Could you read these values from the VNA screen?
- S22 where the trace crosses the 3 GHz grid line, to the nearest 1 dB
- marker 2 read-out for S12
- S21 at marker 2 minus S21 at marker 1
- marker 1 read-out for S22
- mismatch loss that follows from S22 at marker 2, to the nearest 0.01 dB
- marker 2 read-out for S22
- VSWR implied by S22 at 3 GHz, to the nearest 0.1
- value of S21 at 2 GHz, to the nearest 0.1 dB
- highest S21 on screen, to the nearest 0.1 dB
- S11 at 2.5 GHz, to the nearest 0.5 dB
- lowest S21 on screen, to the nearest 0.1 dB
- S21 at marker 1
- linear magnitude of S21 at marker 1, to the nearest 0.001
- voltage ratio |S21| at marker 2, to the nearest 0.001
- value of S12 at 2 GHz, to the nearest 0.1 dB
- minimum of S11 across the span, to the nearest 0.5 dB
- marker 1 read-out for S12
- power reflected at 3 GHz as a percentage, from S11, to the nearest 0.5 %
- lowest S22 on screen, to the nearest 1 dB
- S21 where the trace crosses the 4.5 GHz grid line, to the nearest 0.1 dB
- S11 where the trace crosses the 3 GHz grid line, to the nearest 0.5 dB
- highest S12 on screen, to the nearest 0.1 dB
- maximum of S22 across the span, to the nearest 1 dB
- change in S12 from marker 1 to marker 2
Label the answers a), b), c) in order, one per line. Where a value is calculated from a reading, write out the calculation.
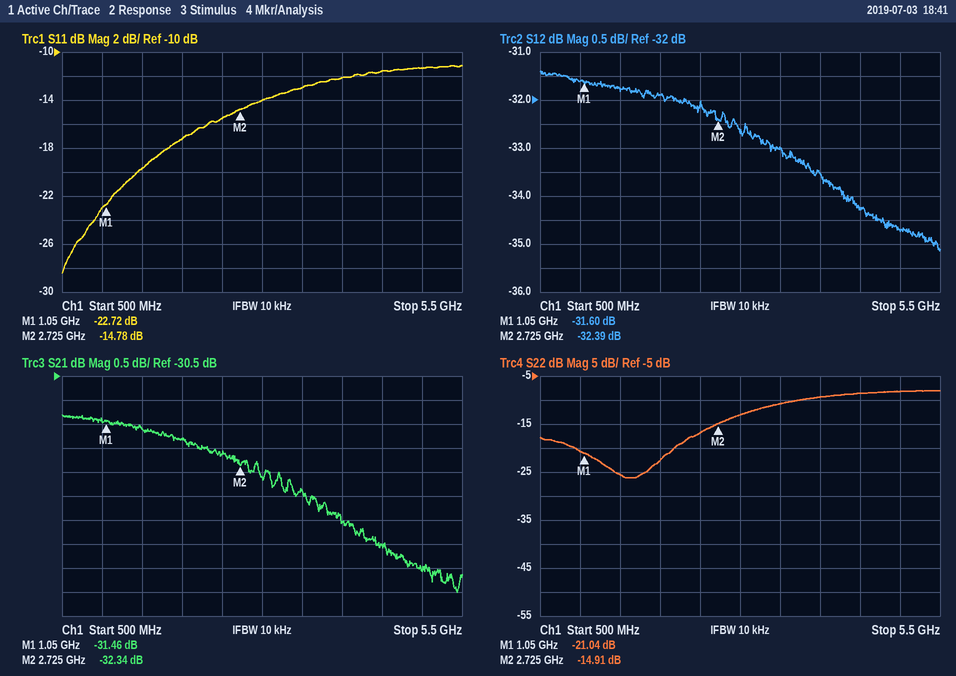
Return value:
a) -13 dB
b) -32.39 dB
c) -32.34 − (-31.46) = -0.88 dB
d) -21.04 dB
e) −10 log10(1 − 10^(-14.91/10)) ≈ 0.14 dB
f) -14.91 dB
g) |Γ| = 10^(-13/20) = 0.2239; VSWR = (1 + 0.2239)/(1 − 0.2239) ≈ 1.6
h) -31.8 dB
i) -31.3 dB
j) -15.5 dB
k) -35.0 dB
l) -31.46 dB
m) 10^(-31.46/20) ≈ 0.027
n) 10^(-32.34/20) ≈ 0.024
o) -31.9 dB
p) -28.5 dB
q) -31.60 dB
r) 10^(-14/10) ≈ 4.0 %
s) -26 dB
t) -34.0 dB
u) -14.0 dB
v) -31.4 dB
w) -8 dB
x) -32.39 − (-31.6) = -0.79 dB
